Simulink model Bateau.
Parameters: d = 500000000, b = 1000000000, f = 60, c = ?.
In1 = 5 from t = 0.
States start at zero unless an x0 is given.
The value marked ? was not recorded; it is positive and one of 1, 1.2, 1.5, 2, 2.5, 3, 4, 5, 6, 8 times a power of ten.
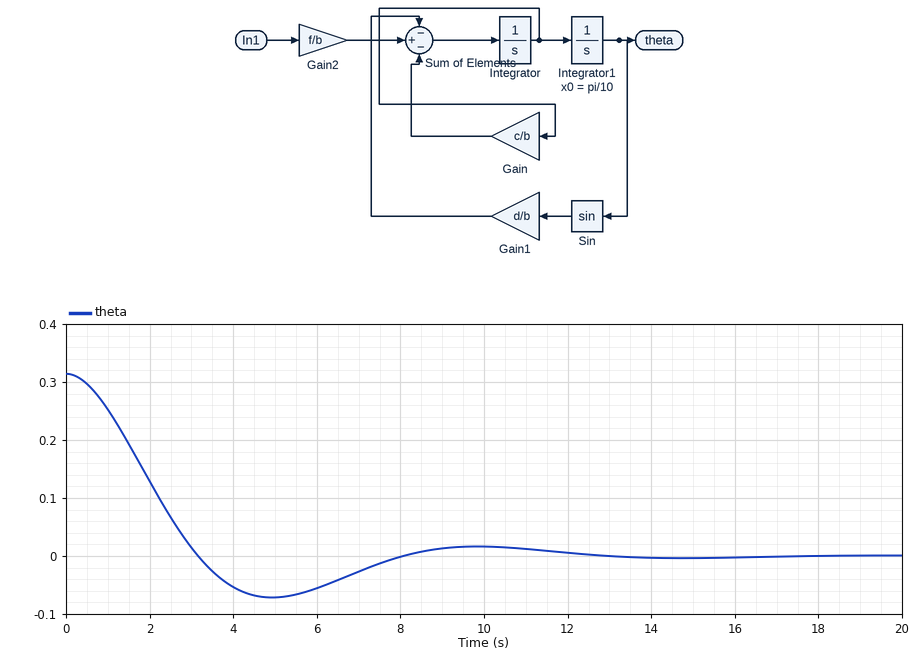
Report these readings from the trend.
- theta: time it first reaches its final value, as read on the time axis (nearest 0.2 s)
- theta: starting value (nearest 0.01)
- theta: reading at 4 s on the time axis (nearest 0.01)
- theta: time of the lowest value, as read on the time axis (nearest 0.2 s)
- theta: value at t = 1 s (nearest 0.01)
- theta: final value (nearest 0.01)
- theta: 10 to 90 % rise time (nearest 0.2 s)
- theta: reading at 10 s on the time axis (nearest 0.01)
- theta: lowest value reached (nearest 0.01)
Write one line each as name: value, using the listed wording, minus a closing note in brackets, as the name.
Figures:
theta: time it first reaches its final value, as read on the time axis: 3.2 s
theta: starting value: 0.31
theta: reading at 4 s on the time axis: -0.05
theta: time of the lowest value, as read on the time axis: 5.0 s
theta: value at t = 1 s: 0.25
theta: final value: 0.00
theta: 10 to 90 % rise time: 2.2 s
theta: reading at 10 s on the time axis: 0.02
theta: lowest value reached: -0.07
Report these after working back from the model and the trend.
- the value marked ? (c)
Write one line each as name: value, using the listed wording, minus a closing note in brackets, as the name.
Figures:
the value marked ?: 6e+08
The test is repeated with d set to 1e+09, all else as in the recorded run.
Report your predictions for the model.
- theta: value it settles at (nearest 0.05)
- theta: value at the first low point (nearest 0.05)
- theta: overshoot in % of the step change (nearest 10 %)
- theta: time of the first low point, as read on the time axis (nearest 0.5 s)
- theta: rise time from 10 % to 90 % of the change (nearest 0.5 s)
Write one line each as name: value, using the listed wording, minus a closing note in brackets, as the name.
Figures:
theta: value it settles at: 0.00
theta: value at the first low point: -0.10
theta: overshoot in % of the step change: 40 %
theta: time of the first low point, as read on the time axis: 3.5 s
theta: rise time from 10 % to 90 % of the change: 1.5 s
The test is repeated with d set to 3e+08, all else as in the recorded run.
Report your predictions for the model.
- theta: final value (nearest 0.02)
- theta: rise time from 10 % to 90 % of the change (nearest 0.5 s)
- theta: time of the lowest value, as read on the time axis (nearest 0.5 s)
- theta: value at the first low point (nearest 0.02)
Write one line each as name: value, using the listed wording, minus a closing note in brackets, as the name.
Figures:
theta: final value: 0.00
theta: rise time from 10 % to 90 % of the change: 3.0 s
theta: time of the lowest value, as read on the time axis: 7.0 s
theta: value at the first low point: -0.04
